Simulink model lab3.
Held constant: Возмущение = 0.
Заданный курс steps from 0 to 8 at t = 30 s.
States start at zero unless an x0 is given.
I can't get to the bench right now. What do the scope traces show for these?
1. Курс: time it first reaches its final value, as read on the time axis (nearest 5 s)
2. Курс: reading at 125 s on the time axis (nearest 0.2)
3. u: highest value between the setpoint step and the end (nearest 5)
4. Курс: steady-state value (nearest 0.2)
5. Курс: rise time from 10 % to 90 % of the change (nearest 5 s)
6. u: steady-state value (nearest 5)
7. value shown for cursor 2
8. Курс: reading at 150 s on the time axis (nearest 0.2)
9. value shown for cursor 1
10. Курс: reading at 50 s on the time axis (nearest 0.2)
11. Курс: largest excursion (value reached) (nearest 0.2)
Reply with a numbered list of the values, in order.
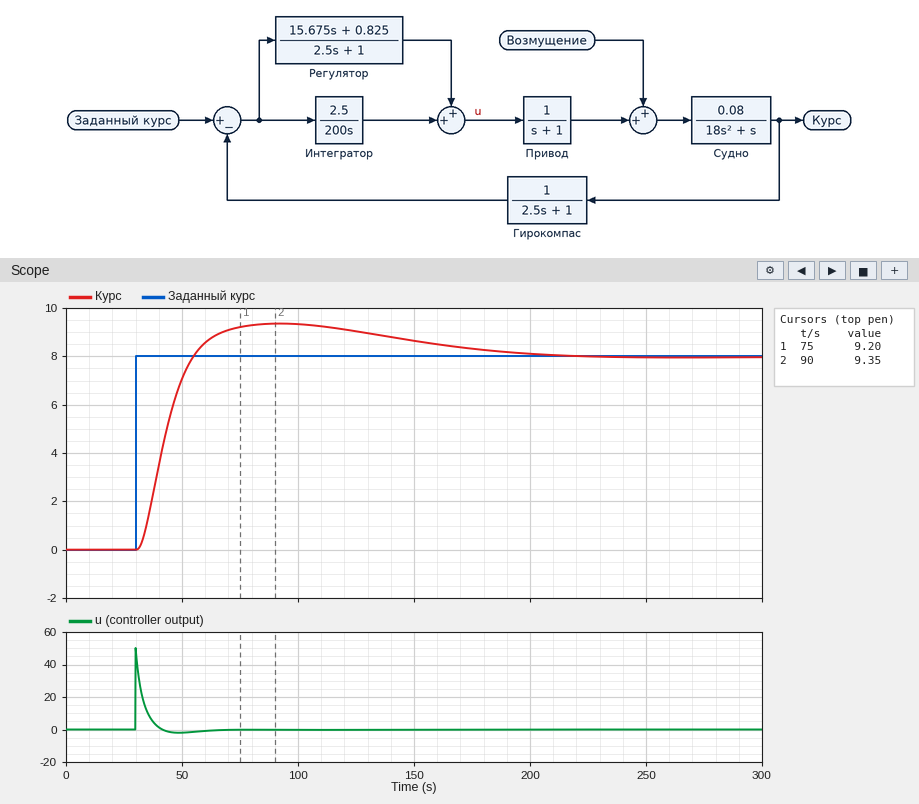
1. 55 s
2. 9.0
3. 50
4. 8.0
5. 15 s
6. 0
7. 9.35
8. 8.6
9. 9.20
10. 7.0
11. 9.4
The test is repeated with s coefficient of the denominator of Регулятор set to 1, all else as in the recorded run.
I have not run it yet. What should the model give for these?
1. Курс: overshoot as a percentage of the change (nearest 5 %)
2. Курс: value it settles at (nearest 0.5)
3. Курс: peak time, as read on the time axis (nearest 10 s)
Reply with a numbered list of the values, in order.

1. 15 %
2. 8.0
3. 100 s
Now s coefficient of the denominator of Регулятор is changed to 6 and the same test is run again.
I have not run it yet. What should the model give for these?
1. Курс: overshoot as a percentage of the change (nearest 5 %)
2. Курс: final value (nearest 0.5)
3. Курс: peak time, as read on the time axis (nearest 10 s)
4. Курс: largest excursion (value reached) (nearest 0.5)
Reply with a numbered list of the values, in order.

1. 25 %
2. 8.0
3. 70 s
4. 10.0
